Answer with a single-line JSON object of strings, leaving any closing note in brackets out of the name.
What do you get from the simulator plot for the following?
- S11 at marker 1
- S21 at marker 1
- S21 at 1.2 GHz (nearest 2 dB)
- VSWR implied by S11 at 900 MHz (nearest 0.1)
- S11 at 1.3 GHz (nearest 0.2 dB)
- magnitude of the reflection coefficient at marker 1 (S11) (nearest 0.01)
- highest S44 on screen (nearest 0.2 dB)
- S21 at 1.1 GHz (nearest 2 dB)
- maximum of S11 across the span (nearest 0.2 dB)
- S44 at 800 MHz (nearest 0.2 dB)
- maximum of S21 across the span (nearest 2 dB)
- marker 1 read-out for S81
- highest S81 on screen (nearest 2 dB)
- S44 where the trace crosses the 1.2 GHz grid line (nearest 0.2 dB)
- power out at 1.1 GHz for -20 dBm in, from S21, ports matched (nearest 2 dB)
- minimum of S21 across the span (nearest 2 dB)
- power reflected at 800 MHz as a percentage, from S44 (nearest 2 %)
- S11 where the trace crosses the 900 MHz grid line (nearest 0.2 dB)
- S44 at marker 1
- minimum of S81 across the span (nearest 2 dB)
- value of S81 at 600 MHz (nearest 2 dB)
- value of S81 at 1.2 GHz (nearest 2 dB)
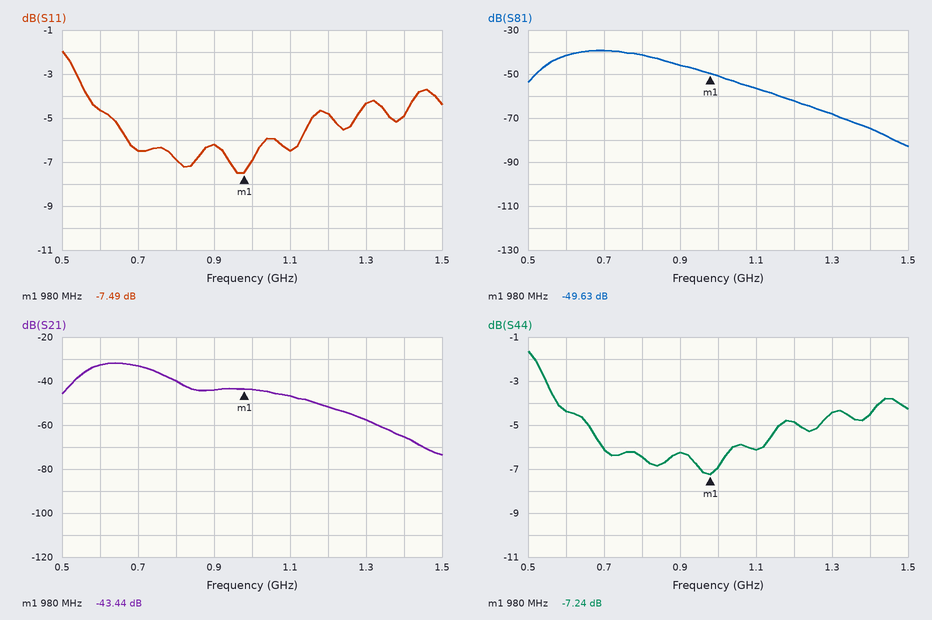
{"S11 at marker 1": "-7.49 dB", "S21 at marker 1": "-43.44 dB", "S21 at 1.2 GHz": "-52 dB", "VSWR implied by S11 at 900 MHz": "2.9", "S11 at 1.3 GHz": "-4.4 dB", "magnitude of the reflection coefficient at marker 1 (S11)": "0.42", "highest S44 on screen": "-1.6 dB", "S21 at 1.1 GHz": "-46 dB", "maximum of S11 across the span": "-2.0 dB", "S44 at 800 MHz": "-6.4 dB", "maximum of S21 across the span": "-32 dB", "marker 1 read-out for S81": "-49.63 dB", "highest S81 on screen": "-40 dB", "S44 where the trace crosses the 1.2 GHz grid line": "-4.8 dB", "power out at 1.1 GHz for -20 dBm in, from S21, ports matched": "-66 dBm", "minimum of S21 across the span": "-74 dB", "power reflected at 800 MHz as a percentage, from S44": "22 %", "S11 where the trace crosses the 900 MHz grid line": "-6.2 dB", "S44 at marker 1": "-7.24 dB", "minimum of S81 across the span": "-82 dB", "value of S81 at 600 MHz": "-42 dB", "value of S81 at 1.2 GHz": "-62 dB"}
